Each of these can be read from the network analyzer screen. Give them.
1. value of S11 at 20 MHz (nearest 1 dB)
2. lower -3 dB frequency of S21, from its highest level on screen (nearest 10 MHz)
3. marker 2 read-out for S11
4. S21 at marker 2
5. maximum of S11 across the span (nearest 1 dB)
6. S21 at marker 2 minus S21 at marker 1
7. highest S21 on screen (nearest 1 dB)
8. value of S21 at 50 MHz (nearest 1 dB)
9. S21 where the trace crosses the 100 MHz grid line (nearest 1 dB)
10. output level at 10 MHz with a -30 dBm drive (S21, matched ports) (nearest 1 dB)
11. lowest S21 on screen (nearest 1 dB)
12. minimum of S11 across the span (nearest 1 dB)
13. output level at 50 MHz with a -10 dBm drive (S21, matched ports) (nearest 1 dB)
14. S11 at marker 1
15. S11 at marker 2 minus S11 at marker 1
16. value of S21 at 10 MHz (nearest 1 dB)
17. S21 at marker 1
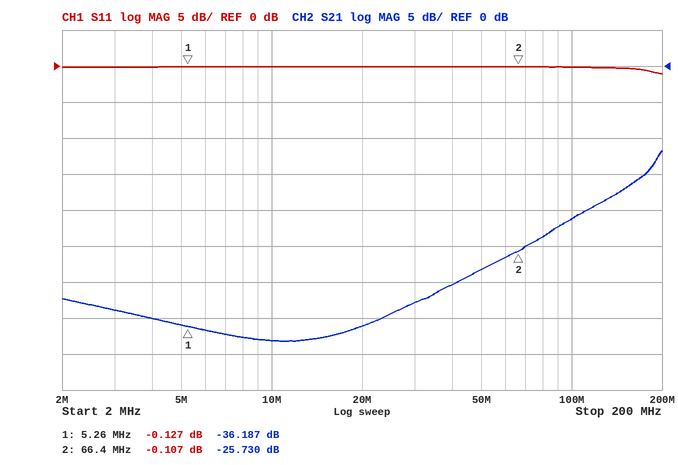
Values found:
0 dB
180 MHz
-0.107 dB
-25.730 dB
0 dB
10.457 dB
-12 dB
-28 dB
-21 dB
-68 dBm
-38 dB
-1 dB
-38 dBm
-0.127 dB
0.020 dB
-38 dB
-36.187 dB
